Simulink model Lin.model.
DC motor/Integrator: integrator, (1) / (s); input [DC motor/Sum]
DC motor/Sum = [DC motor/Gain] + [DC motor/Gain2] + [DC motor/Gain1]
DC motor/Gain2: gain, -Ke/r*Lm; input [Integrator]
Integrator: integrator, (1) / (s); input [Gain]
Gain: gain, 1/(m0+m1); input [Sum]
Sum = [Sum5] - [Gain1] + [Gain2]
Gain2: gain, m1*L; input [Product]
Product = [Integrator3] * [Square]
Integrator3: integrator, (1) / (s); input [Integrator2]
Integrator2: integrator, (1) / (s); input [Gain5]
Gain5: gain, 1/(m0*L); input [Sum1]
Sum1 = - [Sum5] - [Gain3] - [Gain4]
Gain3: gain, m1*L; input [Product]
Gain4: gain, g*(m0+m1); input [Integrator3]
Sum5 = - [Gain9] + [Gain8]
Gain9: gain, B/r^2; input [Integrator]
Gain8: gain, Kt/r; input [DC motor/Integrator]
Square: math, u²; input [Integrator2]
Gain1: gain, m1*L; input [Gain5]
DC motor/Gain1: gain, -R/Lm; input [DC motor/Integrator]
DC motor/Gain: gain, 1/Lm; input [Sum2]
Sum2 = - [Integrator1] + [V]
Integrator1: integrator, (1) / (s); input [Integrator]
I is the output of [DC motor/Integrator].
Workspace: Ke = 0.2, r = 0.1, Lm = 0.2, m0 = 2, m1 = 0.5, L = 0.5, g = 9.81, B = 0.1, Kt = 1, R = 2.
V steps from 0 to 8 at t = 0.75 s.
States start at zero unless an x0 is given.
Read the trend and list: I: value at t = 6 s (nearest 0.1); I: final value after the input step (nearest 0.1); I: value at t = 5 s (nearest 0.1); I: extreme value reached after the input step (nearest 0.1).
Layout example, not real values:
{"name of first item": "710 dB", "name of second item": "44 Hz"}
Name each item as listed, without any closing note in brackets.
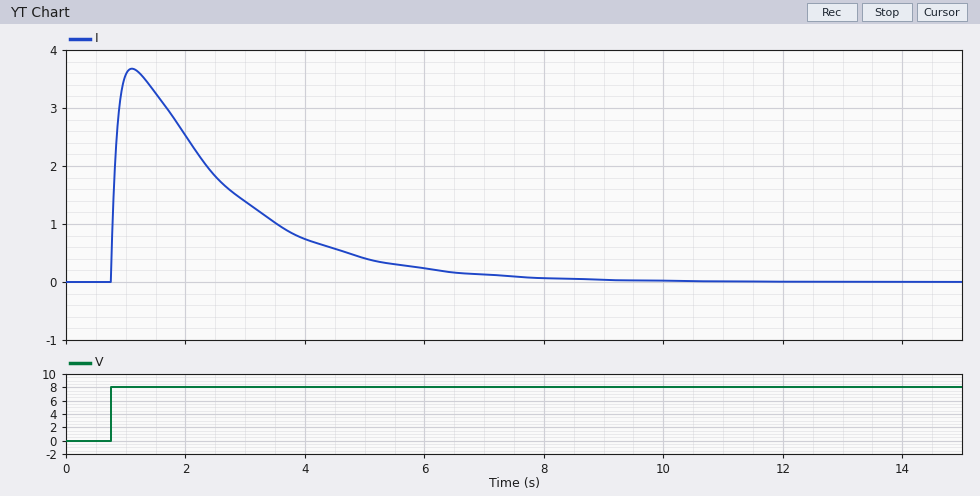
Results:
{"I: value at t = 6 s": "0.2", "I: final value after the input step": "0.0", "I: value at t = 5 s": "0.4", "I: extreme value reached after the input step": "3.7"}
